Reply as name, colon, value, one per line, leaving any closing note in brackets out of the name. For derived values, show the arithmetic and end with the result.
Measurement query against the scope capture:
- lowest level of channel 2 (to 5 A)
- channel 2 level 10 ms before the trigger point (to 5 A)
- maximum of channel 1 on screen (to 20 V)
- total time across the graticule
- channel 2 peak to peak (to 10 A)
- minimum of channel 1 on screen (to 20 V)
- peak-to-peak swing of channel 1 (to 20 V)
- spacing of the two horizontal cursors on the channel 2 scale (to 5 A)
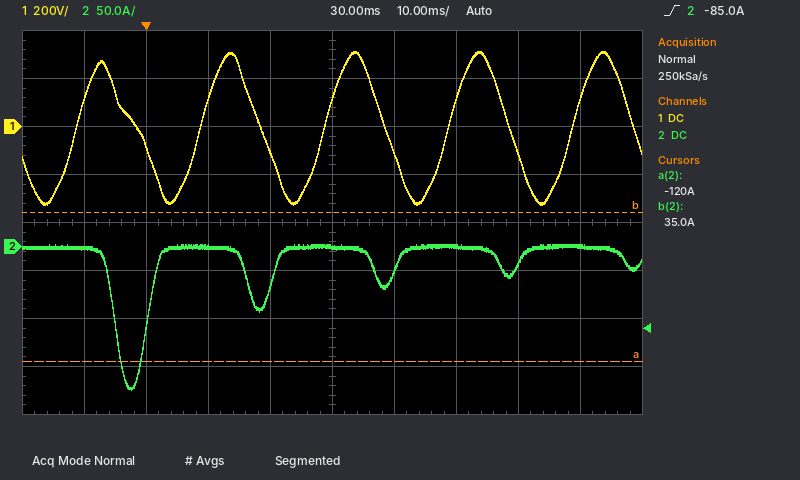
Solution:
lowest level of channel 2: -150 A
channel 2 level 10 ms before the trigger point: 0 A
maximum of channel 1 on screen: 320 V
total time across the graticule: 100 ms
channel 2 peak to peak: 150 A
minimum of channel 1 on screen: -320 V
peak-to-peak swing of channel 1: 320 V − (-320 V) = 640 V
spacing of the two horizontal cursors on the channel 2 scale: 155 A
